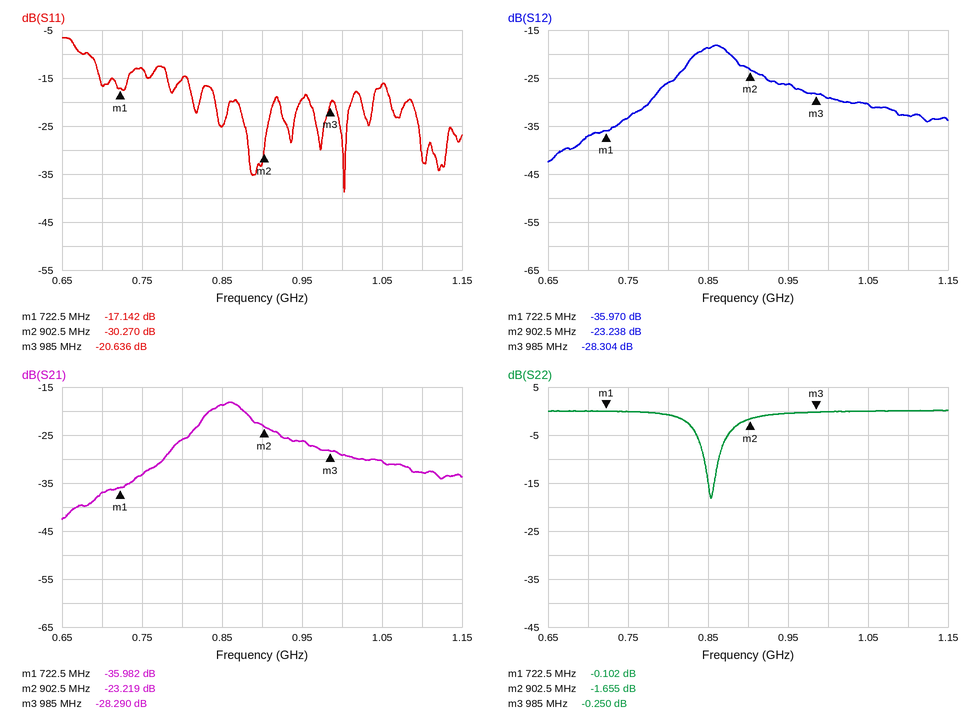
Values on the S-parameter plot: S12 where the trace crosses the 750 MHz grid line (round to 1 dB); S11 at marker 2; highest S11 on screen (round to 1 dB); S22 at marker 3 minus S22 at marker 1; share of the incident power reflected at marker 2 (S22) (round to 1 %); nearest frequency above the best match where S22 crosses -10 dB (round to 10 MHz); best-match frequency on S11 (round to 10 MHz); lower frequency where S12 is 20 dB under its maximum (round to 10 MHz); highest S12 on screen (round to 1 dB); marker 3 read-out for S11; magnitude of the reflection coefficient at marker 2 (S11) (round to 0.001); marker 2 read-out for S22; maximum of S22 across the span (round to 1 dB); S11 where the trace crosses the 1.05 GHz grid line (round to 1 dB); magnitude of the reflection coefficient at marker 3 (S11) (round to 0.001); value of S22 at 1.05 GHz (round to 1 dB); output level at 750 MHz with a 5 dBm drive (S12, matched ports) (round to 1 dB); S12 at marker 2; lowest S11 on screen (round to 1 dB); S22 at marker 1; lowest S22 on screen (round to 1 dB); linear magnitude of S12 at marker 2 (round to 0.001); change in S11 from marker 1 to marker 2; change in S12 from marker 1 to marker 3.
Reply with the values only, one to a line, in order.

-33 dB
-30.270 dB
-7 dB
-0.148 dB
68 %
860 MHz
1.00 GHz
690 MHz
-18 dB
-20.636 dB
0.031
-1.655 dB
0 dB
-16 dB
0.093
0 dB
-28 dBm
-23.238 dB
-39 dB
-0.102 dB
-18 dB
0.069
-13.128 dB
7.666 dB
